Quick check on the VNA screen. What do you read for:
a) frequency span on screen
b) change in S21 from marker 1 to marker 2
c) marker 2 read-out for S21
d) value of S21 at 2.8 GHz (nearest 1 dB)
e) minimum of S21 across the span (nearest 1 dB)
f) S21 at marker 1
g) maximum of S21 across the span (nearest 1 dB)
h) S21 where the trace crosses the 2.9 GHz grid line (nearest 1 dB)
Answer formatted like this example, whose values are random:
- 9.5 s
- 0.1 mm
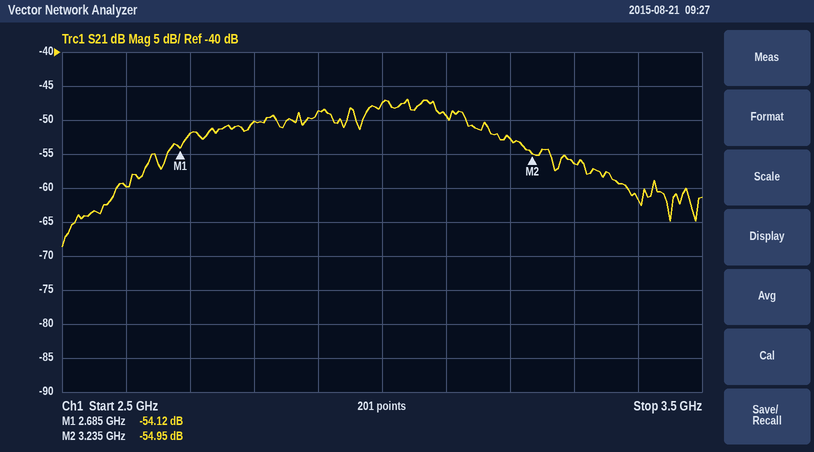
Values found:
- 1 GHz
- -0.83 dB
- -54.95 dB
- -50 dB
- -69 dB
- -54.12 dB
- -47 dB
- -49 dB
